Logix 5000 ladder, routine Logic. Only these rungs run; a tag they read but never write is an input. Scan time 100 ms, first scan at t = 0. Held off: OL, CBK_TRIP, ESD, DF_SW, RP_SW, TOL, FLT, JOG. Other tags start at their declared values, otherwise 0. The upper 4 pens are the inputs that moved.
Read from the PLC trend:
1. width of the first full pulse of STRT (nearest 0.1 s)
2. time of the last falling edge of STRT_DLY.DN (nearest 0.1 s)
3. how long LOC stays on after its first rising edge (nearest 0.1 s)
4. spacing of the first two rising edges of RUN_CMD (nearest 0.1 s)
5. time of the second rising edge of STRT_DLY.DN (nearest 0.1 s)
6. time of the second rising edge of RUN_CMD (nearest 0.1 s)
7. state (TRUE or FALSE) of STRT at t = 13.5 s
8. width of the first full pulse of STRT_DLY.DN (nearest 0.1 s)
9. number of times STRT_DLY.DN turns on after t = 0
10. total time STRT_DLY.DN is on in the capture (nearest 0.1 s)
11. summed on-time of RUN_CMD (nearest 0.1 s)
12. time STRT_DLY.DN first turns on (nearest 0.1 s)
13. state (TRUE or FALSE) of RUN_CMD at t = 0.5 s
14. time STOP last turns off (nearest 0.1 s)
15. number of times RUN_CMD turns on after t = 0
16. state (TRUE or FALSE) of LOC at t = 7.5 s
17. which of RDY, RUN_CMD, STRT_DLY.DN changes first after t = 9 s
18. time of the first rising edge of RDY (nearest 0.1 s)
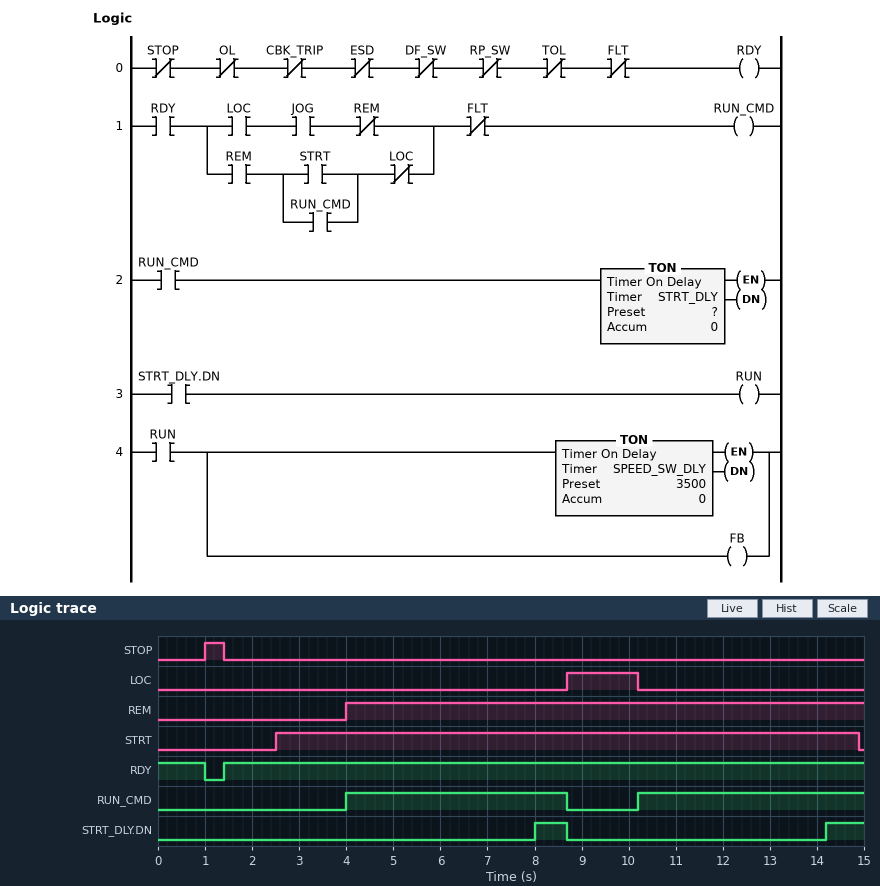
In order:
12.4 s
8.7 s
1.5 s
6.2 s
14.2 s
10.2 s
TRUE
0.7 s
2
1.5 s
9.5 s
8.0 s
FALSE
1.4 s
2
FALSE
RUN_CMD
1.4 s
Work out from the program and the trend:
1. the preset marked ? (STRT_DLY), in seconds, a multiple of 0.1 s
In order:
4.0 s
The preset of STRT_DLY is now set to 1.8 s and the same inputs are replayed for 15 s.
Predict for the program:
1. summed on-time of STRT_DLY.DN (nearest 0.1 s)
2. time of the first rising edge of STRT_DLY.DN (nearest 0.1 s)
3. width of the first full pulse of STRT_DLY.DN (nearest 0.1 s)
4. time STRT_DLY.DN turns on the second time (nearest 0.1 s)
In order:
5.9 s
5.8 s
2.9 s
12.0 s
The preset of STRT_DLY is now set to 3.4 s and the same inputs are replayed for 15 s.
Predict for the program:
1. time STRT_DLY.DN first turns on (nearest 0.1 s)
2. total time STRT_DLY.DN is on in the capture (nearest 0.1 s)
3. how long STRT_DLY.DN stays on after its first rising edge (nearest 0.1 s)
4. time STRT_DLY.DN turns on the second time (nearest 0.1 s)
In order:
7.4 s
2.7 s
1.3 s
13.6 s
